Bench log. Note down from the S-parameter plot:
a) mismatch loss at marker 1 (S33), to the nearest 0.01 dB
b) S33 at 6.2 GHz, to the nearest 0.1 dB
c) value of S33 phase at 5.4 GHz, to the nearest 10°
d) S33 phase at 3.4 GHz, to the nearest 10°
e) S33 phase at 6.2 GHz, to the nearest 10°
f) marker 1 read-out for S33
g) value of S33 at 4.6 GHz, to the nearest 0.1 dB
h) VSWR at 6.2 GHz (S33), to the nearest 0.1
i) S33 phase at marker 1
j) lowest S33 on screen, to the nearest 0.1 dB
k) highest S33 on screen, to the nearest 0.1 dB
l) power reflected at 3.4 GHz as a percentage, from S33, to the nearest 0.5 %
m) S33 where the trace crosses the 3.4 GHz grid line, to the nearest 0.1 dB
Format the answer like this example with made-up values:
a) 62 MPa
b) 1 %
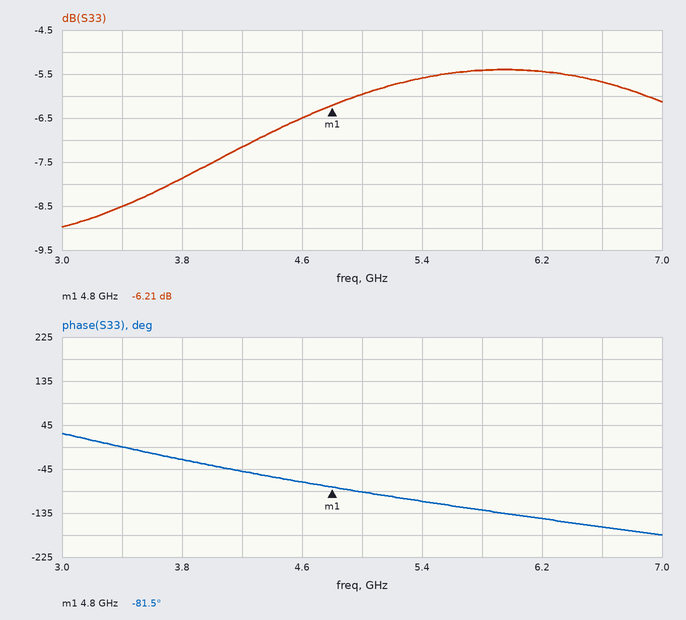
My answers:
a) 1.19 dB
b) -5.4 dB
c) -110°
d) 0°
e) -150°
f) -6.21 dB
g) -6.5 dB
h) 3.3
i) -81.5°
j) -9.0 dB
k) -5.4 dB
l) 14.0 %
m) -8.5 dB
